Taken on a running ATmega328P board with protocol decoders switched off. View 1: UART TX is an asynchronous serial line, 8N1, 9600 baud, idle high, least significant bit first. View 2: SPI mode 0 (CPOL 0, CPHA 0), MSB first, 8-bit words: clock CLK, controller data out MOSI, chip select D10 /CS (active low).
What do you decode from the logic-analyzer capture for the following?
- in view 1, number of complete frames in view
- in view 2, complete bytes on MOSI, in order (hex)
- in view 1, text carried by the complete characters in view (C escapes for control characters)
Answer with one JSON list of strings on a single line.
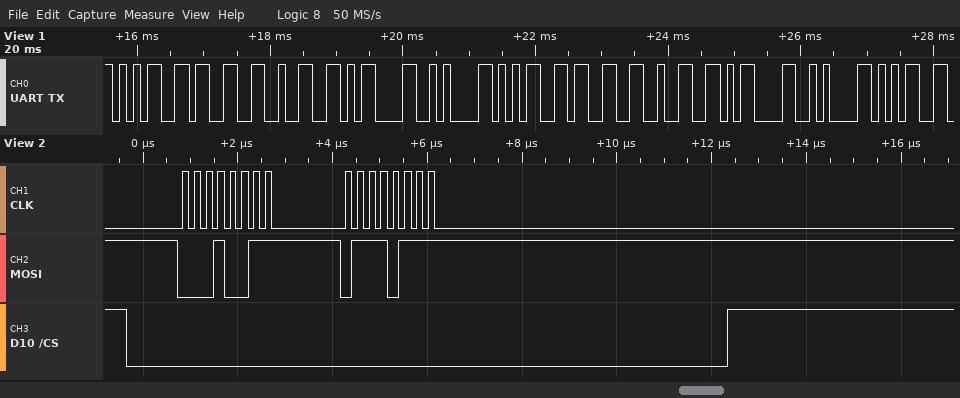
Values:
["11", "13 77", "\"532\\r\\n532\\r\\n5\""]
